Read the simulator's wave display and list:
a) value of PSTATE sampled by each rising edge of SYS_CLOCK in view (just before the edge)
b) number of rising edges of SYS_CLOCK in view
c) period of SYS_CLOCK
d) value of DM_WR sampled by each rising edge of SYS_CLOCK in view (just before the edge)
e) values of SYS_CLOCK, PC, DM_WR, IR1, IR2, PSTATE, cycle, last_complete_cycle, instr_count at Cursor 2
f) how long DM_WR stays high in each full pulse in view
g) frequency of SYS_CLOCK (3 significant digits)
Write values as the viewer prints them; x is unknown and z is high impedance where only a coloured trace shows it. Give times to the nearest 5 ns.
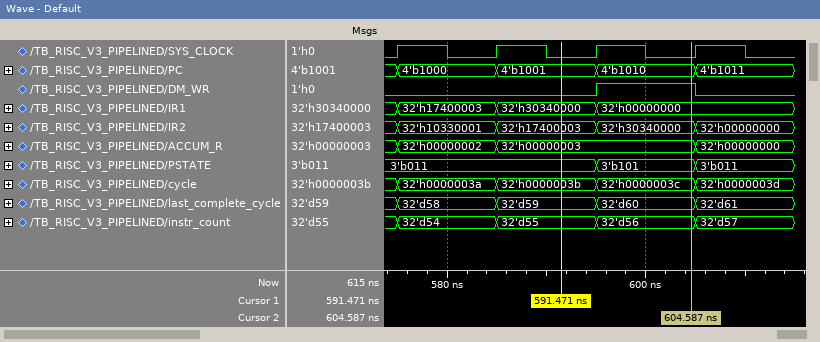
3'b011, 3'b011, 3'b011, 3'b101
4
10 ns
0 0 0 1
SYS_CLOCK=0, PC=4'b1010, DM_WR=1, IR1=32'h00000000, IR2=32'h30340000, PSTATE=3'b101, cycle=32'h0000003c, last_complete_cycle=32'd60, instr_count=32'd56
10 ns
100 MHz
